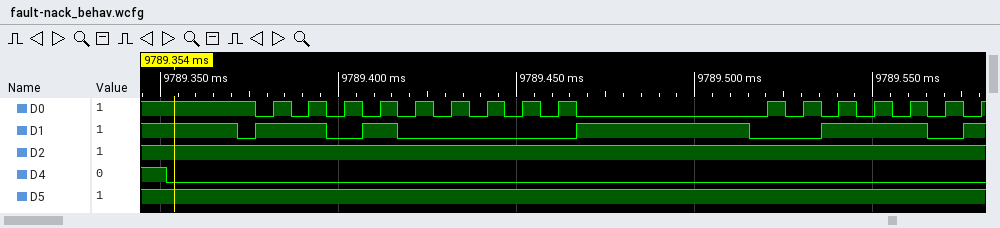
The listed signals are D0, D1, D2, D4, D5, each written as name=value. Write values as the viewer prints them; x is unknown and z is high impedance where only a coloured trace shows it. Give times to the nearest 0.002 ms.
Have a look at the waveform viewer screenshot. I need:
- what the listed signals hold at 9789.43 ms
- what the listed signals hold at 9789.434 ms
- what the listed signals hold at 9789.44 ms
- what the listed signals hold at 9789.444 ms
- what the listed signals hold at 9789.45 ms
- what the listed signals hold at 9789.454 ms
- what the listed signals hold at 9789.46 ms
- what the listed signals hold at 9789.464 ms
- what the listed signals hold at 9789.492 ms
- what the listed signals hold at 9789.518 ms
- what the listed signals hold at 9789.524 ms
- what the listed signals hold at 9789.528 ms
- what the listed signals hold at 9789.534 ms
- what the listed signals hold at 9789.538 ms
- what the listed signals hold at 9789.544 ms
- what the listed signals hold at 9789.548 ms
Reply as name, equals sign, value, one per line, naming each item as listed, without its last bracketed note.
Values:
what the listed signals hold at 9789.43 ms = D0=0, D1=0, D2=1, D4=0, D5=1
what the listed signals hold at 9789.434 ms = D0=1, D1=0, D2=1, D4=0, D5=1
what the listed signals hold at 9789.44 ms = D0=0, D1=0, D2=1, D4=0, D5=1
what the listed signals hold at 9789.444 ms = D0=1, D1=0, D2=1, D4=0, D5=1
what the listed signals hold at 9789.45 ms = D0=0, D1=0, D2=1, D4=0, D5=1
what the listed signals hold at 9789.454 ms = D0=1, D1=0, D2=1, D4=0, D5=1
what the listed signals hold at 9789.46 ms = D0=0, D1=0, D2=1, D4=0, D5=1
what the listed signals hold at 9789.464 ms = D0=1, D1=0, D2=1, D4=0, D5=1
what the listed signals hold at 9789.492 ms = D0=0, D1=1, D2=1, D4=0, D5=1
what the listed signals hold at 9789.518 ms = D0=0, D1=0, D2=1, D4=0, D5=1
what the listed signals hold at 9789.524 ms = D0=1, D1=0, D2=1, D4=0, D5=1
what the listed signals hold at 9789.528 ms = D0=0, D1=0, D2=1, D4=0, D5=1
what the listed signals hold at 9789.534 ms = D0=1, D1=0, D2=1, D4=0, D5=1
what the listed signals hold at 9789.538 ms = D0=0, D1=1, D2=1, D4=0, D5=1
what the listed signals hold at 9789.544 ms = D0=1, D1=1, D2=1, D4=0, D5=1
what the listed signals hold at 9789.548 ms = D0=0, D1=1, D2=1, D4=0, D5=1
